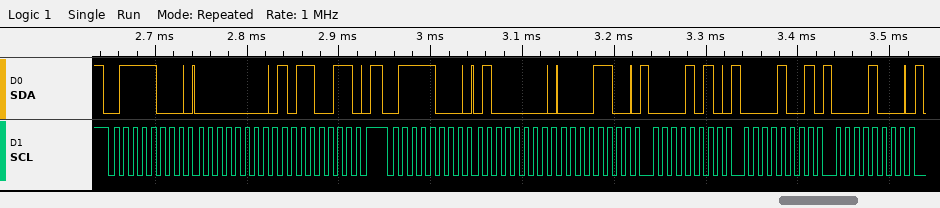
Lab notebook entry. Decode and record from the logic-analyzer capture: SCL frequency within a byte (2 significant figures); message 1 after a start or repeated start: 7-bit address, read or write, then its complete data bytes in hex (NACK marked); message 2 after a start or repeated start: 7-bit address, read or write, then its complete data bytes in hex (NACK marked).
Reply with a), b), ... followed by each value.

a) 100 kHz
b) 0x3C write: 00 B3
c) 0x3C write: 40 0C 0A 09 08
